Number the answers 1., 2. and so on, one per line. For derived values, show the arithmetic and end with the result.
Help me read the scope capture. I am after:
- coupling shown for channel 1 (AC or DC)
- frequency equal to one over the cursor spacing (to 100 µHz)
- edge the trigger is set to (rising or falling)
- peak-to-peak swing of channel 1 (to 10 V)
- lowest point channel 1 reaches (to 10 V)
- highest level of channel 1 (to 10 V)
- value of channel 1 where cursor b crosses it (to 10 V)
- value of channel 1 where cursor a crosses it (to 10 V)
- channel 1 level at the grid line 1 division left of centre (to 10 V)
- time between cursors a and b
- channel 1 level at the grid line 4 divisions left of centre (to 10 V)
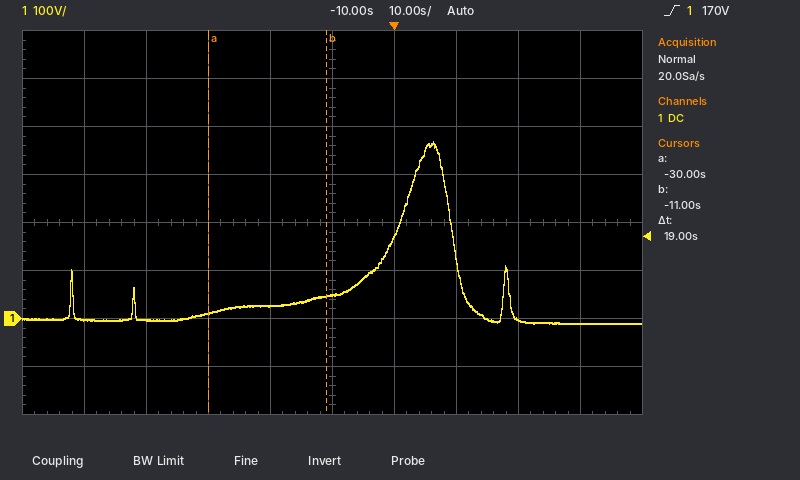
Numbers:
1. DC
2. 1 / 19 s ≈ 52.6 mHz
3. rising
4. 370 V − (-10 V) = 380 V
5. -10 V
6. 370 V
7. 50 V
8. 10 V
9. 30 V
10. 19 s
11. 0 V
